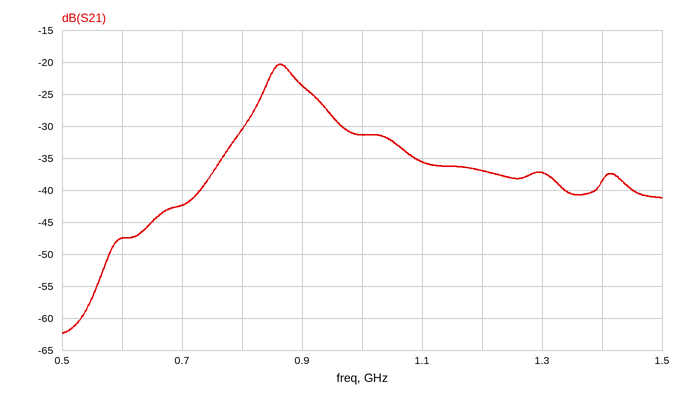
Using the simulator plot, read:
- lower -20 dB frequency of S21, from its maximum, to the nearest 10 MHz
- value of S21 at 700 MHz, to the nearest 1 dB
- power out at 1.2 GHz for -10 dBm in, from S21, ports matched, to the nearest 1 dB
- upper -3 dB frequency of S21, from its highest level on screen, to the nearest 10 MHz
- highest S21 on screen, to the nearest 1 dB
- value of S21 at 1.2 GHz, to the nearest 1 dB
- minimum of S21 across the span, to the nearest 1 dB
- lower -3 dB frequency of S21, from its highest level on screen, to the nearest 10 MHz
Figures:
730 MHz
-42 dB
-47 dBm
900 MHz
-20 dB
-37 dB
-62 dB
840 MHz
